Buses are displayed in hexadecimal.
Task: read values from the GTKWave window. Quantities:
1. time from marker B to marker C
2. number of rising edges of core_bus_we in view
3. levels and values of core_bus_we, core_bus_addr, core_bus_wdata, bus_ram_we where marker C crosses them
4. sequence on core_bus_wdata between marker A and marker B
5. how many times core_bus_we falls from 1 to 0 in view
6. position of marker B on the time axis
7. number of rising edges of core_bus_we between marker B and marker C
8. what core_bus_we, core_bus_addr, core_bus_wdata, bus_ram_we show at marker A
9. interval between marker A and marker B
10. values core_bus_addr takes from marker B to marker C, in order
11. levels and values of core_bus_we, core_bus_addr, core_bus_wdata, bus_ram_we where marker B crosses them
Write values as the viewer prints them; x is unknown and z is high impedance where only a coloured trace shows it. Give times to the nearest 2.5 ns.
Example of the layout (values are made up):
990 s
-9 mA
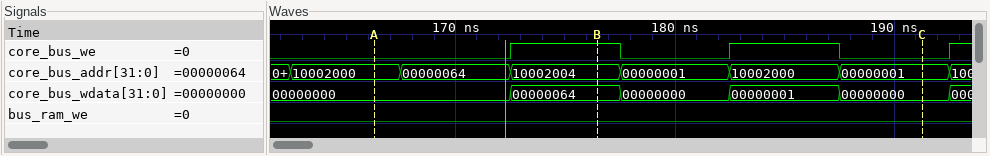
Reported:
15 ns
3
core_bus_we=0, core_bus_addr=00000001, core_bus_wdata=00000000, bus_ram_we=0
00000000, 00000064
2
177.5 ns
1
core_bus_we=0, core_bus_addr=10002000, core_bus_wdata=00000000, bus_ram_we=0
10 ns
10002004, 00000001, 10002000, 00000001
core_bus_we=1, core_bus_addr=10002004, core_bus_wdata=00000064, bus_ram_we=0
